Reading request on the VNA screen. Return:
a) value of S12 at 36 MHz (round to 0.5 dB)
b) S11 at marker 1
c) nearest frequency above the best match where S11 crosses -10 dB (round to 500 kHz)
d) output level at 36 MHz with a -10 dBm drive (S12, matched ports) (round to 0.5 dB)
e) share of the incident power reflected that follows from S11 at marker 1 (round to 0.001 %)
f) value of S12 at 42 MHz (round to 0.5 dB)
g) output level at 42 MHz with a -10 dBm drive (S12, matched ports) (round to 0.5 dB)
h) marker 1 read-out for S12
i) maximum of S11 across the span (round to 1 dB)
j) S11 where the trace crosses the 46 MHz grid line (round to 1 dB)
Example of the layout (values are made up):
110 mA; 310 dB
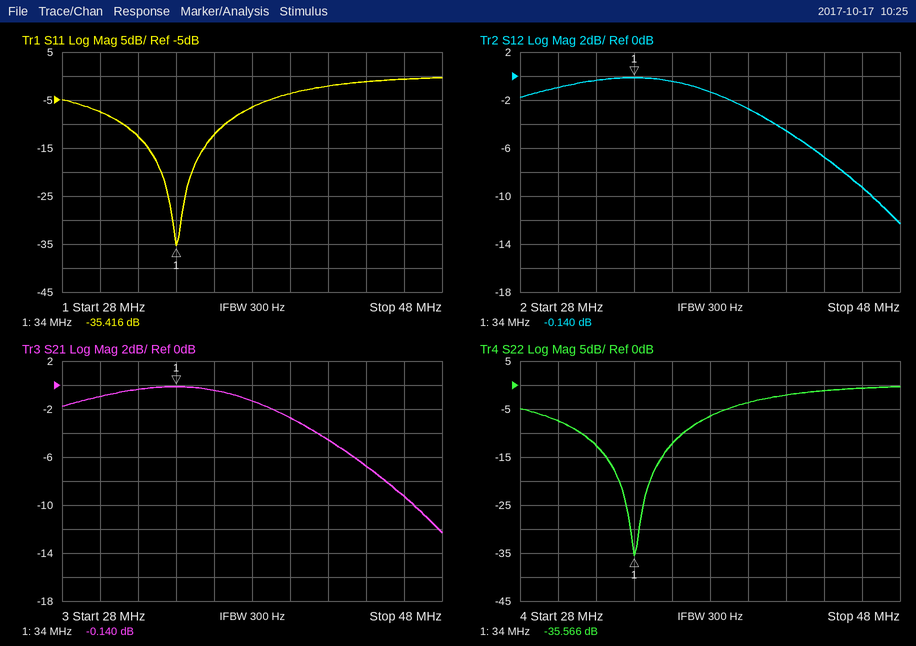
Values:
-0.5 dB; -35.416 dB; 36.5 MHz; -10.5 dBm; 0.029 %; -4.5 dB; -14.5 dBm; -0.140 dB; 0 dB; -1 dB
